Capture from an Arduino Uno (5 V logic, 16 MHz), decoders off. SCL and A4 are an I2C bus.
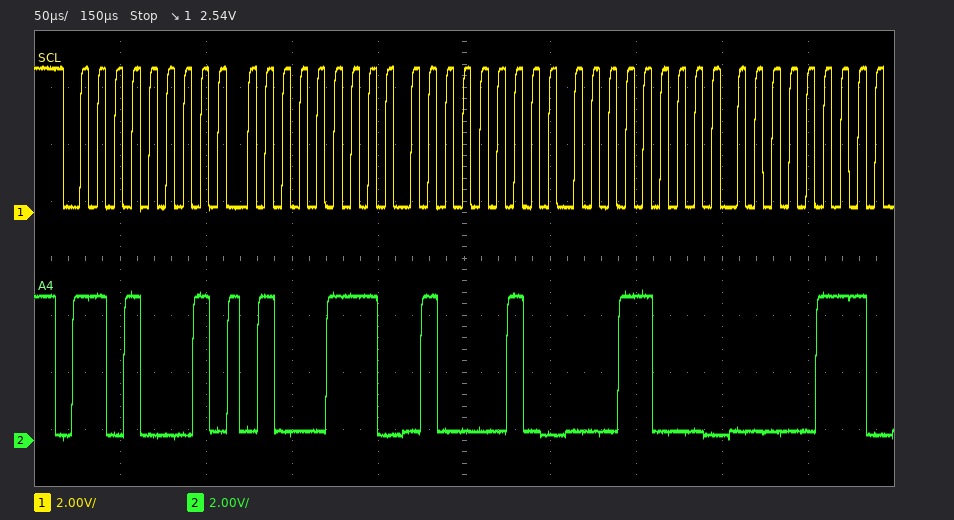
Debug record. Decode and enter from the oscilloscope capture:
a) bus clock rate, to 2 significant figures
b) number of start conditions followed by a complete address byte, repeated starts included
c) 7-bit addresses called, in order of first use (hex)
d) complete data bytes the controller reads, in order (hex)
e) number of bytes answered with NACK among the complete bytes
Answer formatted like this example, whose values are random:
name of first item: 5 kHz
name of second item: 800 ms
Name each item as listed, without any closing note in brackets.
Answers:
bus clock rate, to 2 significant figures: 100 kHz
number of start conditions followed by a complete address byte, repeated starts included: 1
7-bit addresses called, in order of first use: 0x68
complete data bytes the controller reads, in order: 47 42 18 07
number of bytes answered with NACK among the complete bytes: 0
